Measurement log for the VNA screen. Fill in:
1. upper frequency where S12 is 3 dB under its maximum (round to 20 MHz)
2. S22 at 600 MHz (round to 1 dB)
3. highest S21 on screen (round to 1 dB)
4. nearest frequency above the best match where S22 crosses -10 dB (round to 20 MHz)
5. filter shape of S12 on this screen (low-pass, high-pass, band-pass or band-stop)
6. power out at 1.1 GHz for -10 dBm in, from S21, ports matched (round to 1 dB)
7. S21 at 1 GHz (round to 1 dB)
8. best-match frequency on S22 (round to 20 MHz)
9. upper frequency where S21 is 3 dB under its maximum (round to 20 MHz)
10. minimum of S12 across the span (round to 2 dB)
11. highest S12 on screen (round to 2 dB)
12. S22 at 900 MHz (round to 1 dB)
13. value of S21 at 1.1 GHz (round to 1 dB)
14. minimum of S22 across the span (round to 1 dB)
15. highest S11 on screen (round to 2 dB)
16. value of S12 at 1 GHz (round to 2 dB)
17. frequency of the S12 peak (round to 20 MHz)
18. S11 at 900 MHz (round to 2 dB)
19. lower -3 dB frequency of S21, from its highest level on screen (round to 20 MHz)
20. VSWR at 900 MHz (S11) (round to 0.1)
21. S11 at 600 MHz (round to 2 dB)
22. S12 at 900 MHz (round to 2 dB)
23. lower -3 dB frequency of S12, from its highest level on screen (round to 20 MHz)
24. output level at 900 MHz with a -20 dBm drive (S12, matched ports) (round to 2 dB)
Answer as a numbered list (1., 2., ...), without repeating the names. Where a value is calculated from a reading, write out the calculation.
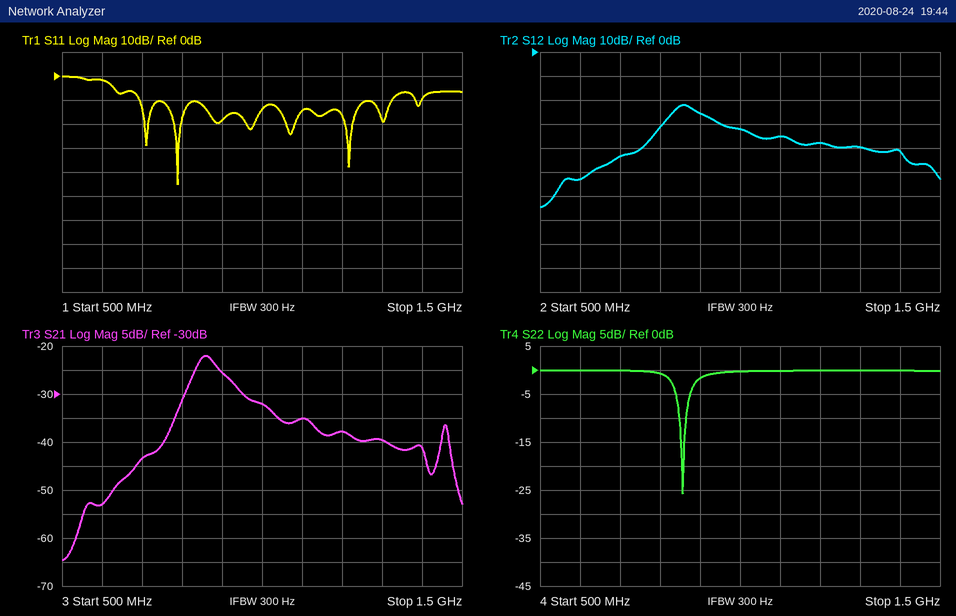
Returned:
1. 900 MHz
2. 0 dB
3. -22 dB
4. 860 MHz
5. band-pass
6. -10 dBm + (-35 dB) = -45 dBm
7. -32 dB
8. 860 MHz
9. 900 MHz
10. -64 dB
11. -22 dB
12. -2 dB
13. -35 dB
14. -26 dB
15. 0 dB
16. -32 dB
17. 860 MHz
18. -18 dB
19. 840 MHz
20. |Γ| = 10^(-18/20) = 0.1259; VSWR = (1 + 0.1259)/(1 − 0.1259) ≈ 1.3
21. -2 dB
22. -26 dB
23. 840 MHz
24. -20 dBm + (-26 dB) = -46 dBm
